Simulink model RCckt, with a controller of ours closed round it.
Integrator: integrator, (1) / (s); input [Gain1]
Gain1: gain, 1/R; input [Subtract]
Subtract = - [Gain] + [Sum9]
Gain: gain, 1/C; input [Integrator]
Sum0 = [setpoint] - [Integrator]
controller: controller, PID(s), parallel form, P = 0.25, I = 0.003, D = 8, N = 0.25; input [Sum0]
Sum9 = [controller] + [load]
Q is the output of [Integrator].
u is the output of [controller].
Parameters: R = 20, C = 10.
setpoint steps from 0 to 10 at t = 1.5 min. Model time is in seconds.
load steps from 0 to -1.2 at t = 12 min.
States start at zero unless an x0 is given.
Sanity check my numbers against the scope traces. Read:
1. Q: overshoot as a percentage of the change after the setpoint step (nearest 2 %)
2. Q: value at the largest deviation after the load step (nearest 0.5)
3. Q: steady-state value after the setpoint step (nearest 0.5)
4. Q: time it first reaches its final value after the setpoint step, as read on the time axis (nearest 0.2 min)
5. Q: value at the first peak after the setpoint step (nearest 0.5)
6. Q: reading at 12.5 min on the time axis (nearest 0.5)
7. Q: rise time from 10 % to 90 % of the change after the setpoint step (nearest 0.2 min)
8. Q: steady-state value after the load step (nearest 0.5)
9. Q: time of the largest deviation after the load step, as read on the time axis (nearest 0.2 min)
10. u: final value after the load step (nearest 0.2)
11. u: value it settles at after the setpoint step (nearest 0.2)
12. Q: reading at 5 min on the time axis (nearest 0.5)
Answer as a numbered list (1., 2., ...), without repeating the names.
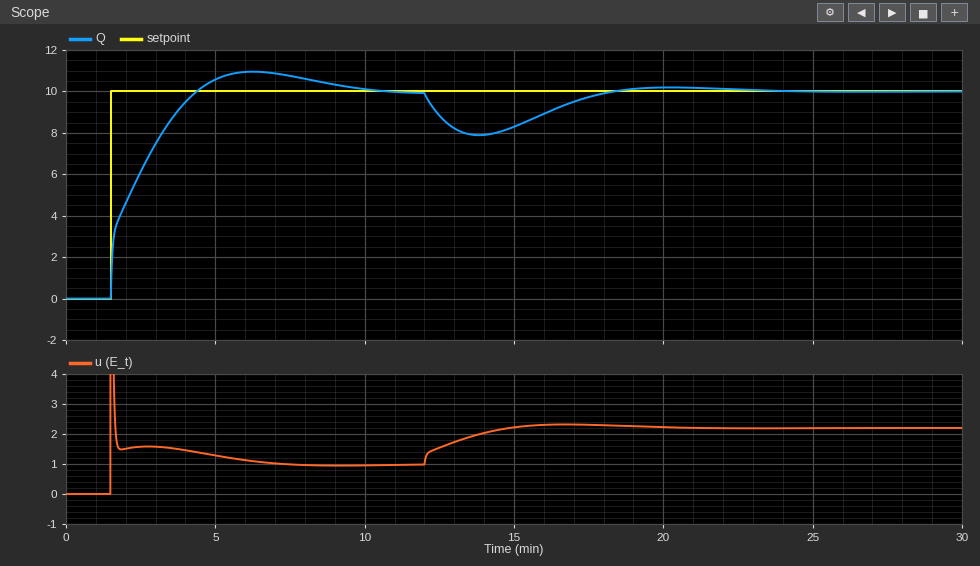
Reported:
1. 10 %
2. 8.0
3. 10.0
4. 4.4 min
5. 11.0
6. 9.0
7. 2.2 min
8. 10.0
9. 13.8 min
10. 2.2
11. 1.0
12. 10.5
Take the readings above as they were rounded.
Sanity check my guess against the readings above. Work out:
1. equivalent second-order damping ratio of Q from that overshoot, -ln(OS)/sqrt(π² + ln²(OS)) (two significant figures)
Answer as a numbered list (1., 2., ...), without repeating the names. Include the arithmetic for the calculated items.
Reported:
1. ln(0.1) = -2.303; 2.303 / sqrt(9.870 + 5.302) = 0.59
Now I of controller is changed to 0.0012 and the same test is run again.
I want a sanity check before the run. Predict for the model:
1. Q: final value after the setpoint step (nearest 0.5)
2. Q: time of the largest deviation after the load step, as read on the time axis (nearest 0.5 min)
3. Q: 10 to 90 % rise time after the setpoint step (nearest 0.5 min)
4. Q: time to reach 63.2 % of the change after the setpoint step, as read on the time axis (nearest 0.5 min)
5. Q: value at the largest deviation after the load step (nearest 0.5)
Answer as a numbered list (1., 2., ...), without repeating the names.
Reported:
1. 10.0
2. 14.5 min
3. 4.0 min
4. 3.0 min
5. 7.5
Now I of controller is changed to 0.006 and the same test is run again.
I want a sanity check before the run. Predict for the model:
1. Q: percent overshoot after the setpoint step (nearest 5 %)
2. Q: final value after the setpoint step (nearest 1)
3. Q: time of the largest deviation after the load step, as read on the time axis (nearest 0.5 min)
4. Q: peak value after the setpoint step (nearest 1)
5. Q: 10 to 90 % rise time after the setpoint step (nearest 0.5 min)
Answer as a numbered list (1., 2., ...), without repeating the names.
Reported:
1. 20 %
2. 10
3. 13.5 min
4. 12
5. 1.5 min
